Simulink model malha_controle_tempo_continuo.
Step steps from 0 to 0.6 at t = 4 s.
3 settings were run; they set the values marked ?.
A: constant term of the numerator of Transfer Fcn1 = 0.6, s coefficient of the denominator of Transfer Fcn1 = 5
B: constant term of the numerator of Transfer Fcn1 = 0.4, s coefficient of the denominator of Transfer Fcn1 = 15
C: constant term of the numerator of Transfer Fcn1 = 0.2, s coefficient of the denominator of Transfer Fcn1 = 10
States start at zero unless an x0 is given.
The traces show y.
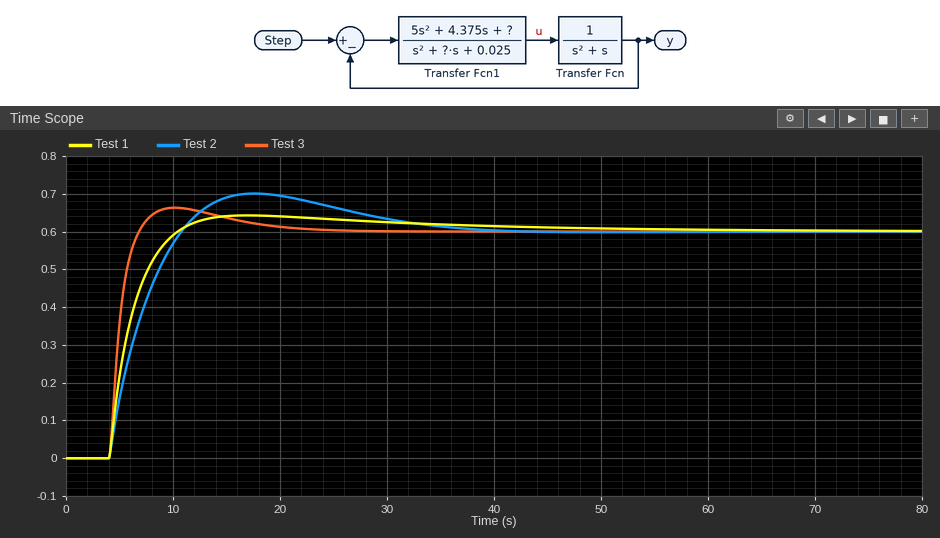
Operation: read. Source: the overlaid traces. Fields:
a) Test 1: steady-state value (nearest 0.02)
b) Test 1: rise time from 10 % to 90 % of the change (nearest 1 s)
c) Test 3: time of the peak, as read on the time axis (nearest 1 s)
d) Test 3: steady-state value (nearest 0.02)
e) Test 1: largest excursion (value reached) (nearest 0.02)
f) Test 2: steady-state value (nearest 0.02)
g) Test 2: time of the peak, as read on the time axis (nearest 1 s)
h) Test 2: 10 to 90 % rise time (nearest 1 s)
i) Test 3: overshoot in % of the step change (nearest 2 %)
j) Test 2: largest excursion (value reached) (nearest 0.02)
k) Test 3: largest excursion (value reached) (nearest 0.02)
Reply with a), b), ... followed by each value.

a) 0.60
b) 4 s
c) 10 s
d) 0.60
e) 0.64
f) 0.60
g) 18 s
h) 5 s
i) 10 %
j) 0.70
k) 0.66
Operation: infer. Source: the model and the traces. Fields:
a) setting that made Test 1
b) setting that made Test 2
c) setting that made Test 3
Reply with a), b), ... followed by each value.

a) C
b) B
c) A
